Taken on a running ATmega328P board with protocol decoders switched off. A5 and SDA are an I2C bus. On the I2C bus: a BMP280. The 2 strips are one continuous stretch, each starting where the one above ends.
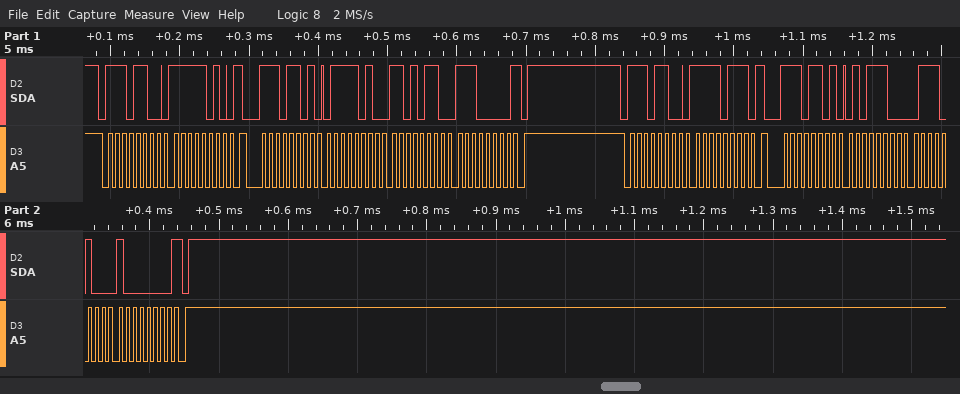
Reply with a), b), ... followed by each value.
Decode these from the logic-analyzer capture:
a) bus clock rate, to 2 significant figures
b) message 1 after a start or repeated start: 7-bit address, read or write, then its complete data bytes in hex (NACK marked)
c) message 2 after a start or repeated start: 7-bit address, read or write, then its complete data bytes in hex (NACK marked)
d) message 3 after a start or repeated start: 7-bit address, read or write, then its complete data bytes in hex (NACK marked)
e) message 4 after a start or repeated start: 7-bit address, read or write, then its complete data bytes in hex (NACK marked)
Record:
a) 100 kHz
b) 0x76 write: FA
c) 0x76 read: 7A D6 E0 NACK
d) 0x76 write: F7
e) 0x76 read: 5C 74 80 NACK
